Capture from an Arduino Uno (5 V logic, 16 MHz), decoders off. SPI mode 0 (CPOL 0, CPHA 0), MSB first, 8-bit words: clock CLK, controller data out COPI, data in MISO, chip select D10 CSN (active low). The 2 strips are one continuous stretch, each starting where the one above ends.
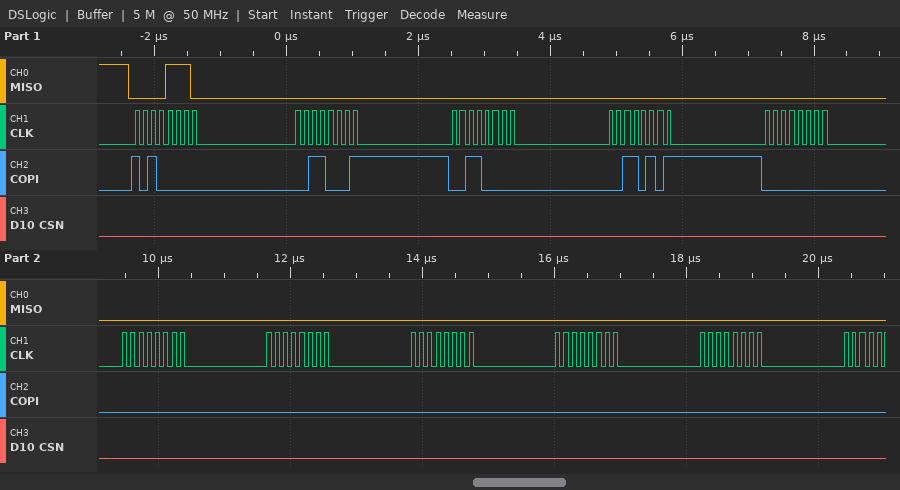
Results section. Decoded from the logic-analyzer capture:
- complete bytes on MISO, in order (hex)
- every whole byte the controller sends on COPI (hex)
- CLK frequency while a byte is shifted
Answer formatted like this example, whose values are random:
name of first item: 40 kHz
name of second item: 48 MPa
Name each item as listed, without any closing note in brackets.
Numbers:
complete bytes on MISO, in order: 0E 00 00 00 00 00 00 00 00 00
every whole byte the controller sends on COPI: A0 31 30 35 00 00 00 00 00 00
CLK frequency while a byte is shifted: 8 MHz
